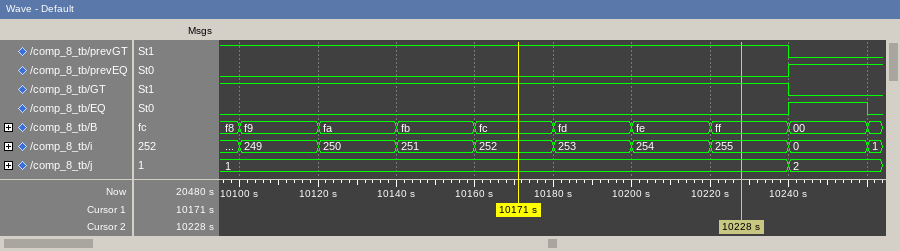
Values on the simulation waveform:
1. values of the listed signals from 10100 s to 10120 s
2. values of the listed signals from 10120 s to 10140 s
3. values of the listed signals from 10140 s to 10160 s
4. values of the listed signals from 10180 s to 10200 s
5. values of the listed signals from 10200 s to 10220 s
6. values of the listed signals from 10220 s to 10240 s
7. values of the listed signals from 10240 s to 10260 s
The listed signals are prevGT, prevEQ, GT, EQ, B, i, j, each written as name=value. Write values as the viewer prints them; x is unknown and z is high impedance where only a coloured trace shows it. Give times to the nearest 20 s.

prevGT=1, prevEQ=0, GT=1, EQ=0, B=f9, i=249, j=1
prevGT=1, prevEQ=0, GT=1, EQ=0, B=fa, i=250, j=1
prevGT=1, prevEQ=0, GT=1, EQ=0, B=fb, i=251, j=1
prevGT=1, prevEQ=0, GT=1, EQ=0, B=fd, i=253, j=1
prevGT=1, prevEQ=0, GT=1, EQ=0, B=fe, i=254, j=1
prevGT=1, prevEQ=0, GT=1, EQ=0, B=ff, i=255, j=1
prevGT=0, prevEQ=1, GT=0, EQ=1, B=00, i=0, j=2
